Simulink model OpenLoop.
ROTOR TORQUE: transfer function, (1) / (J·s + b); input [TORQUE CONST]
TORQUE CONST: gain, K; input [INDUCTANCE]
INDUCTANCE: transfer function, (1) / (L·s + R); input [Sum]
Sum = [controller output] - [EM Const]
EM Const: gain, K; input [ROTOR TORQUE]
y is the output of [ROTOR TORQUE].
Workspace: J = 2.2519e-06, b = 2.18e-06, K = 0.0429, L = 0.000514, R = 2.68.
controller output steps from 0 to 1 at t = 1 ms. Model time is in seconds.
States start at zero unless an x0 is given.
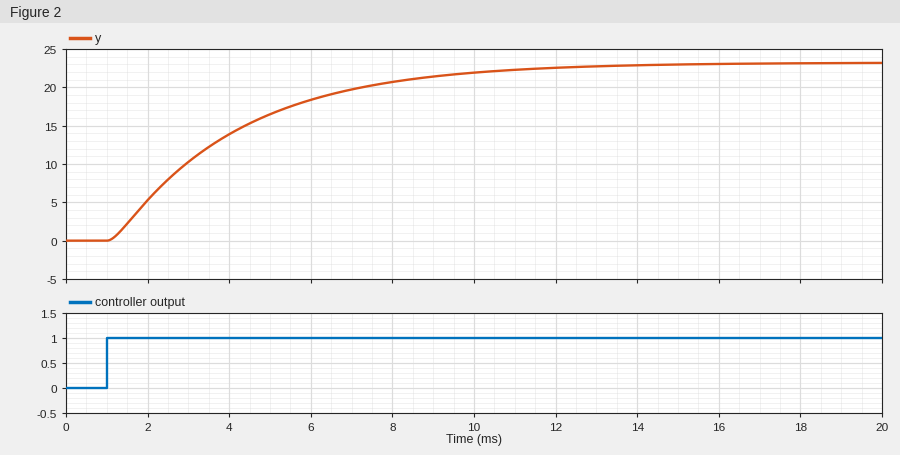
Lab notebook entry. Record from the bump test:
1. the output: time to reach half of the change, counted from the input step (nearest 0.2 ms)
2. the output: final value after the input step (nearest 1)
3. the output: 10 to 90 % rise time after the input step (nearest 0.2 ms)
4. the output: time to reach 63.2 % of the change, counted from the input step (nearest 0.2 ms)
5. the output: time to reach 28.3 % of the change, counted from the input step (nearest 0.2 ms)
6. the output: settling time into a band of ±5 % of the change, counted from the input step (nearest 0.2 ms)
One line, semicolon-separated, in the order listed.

2.4 ms; 23; 6.8 ms; 3.2 ms; 1.2 ms; 9.4 ms
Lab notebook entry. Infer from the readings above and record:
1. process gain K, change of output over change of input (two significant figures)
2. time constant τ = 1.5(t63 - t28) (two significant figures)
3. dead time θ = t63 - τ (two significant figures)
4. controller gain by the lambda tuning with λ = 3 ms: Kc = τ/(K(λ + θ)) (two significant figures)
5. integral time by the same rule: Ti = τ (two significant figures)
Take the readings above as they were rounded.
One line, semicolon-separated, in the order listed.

23; 3.0 ms; 0.20 ms; 0.041; 3.0 ms
